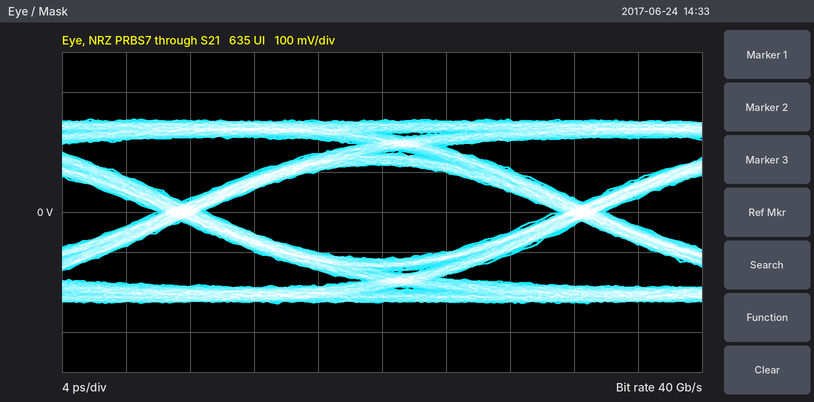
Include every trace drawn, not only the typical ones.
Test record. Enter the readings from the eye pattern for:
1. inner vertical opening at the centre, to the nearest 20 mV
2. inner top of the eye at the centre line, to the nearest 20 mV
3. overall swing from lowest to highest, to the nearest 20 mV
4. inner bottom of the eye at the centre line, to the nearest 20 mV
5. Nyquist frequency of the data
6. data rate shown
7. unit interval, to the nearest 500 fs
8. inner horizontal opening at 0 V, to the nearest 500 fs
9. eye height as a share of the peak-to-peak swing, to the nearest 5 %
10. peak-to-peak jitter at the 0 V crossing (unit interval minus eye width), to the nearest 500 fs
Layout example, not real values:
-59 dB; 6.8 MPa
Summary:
240 mV; 120 mV; 460 mV; -120 mV; 20 GHz; 40 Gb/s; 25.0 ps; 22.0 ps; 50 %; 3.0 ps
